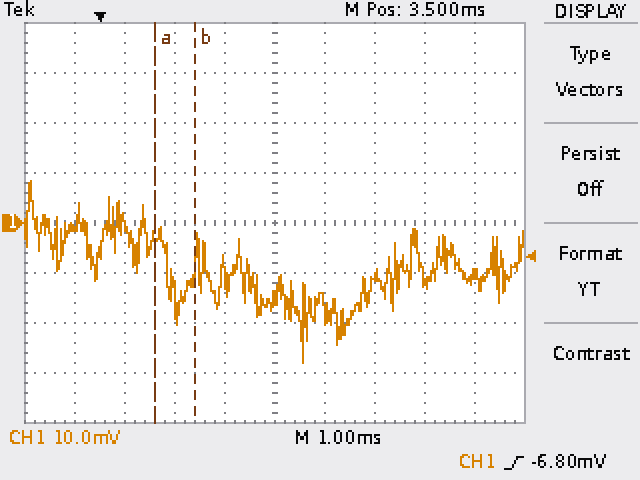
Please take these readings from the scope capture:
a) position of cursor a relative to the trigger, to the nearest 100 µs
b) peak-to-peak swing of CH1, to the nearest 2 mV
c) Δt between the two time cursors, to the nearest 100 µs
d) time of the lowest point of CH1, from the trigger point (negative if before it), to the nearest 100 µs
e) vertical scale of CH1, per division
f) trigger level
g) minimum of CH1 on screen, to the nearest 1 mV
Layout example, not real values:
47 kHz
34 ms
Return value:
+1.1 ms
36 mV
800 µs
+4.1 ms
10 mV
-6.80 mV
-28 mV
